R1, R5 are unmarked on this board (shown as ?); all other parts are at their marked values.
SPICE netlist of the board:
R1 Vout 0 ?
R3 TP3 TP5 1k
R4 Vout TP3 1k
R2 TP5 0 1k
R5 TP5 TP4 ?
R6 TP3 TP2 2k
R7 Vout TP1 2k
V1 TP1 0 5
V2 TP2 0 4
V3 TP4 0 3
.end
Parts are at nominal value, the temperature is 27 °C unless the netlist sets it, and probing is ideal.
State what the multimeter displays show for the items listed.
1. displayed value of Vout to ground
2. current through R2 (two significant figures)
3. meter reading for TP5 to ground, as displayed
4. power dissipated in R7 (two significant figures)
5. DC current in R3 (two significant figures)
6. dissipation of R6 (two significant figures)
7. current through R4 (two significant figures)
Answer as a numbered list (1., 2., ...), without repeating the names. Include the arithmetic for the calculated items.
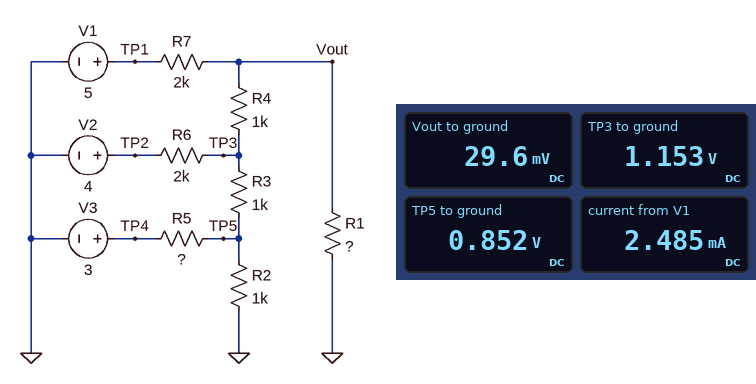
1. 29.6 mV
2. (852 mV) / 1 kΩ = 850 µA
3. 0.852 V
4. (5 V - 29.6 mV)^2 / 2 kΩ = 12 mW
5. (1.153 V - 852 mV) / 1 kΩ = 300 µA
6. (4 V - 1.153 V)^2 / 2 kΩ = 4.1 mW
7. (1.153 V - 29.6 mV) / 1 kΩ = 1.1 mA
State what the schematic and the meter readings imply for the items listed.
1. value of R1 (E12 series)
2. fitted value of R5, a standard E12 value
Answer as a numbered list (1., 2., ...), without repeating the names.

1. 8.2 Ω
2. 3.9 kΩ
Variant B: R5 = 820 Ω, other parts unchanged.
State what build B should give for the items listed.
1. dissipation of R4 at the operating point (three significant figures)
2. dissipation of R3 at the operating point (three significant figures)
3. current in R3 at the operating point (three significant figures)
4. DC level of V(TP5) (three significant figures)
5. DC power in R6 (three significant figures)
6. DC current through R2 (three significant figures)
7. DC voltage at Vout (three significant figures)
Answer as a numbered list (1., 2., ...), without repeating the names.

1. 2.00 mW
2. 19.2 µW
3. 139 µA
4. 1.59 V
5. 3.26 mW
6. 1.59 mA
7. 32.0 mV
